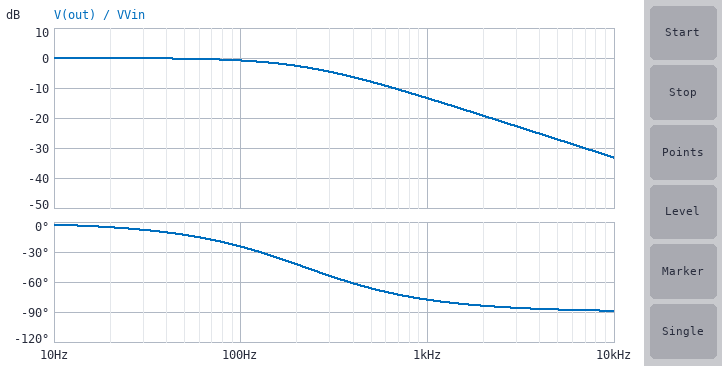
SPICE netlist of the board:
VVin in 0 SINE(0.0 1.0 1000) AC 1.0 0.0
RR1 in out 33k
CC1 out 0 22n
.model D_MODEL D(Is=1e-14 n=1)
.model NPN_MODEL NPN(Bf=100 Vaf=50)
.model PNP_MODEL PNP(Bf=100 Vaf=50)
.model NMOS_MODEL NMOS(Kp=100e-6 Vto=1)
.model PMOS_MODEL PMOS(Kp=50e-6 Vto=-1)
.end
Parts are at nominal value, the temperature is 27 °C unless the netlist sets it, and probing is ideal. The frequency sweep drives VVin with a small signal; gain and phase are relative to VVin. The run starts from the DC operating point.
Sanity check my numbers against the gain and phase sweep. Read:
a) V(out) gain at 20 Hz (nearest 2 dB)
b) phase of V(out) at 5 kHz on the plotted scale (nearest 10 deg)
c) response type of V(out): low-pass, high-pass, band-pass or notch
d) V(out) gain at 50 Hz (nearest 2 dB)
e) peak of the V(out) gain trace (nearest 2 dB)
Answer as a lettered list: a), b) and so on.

a) 0 dB
b) -90 deg
c) low-pass
d) 0 dB
e) 0 dB
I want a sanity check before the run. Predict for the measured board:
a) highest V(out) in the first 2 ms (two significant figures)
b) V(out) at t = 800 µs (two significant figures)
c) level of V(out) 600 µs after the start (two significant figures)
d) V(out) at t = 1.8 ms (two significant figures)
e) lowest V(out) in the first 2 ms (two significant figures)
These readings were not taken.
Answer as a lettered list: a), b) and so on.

a) 330 mV
b) -39 mV
c) 230 mV
d) -91 mV
e) -200 mV
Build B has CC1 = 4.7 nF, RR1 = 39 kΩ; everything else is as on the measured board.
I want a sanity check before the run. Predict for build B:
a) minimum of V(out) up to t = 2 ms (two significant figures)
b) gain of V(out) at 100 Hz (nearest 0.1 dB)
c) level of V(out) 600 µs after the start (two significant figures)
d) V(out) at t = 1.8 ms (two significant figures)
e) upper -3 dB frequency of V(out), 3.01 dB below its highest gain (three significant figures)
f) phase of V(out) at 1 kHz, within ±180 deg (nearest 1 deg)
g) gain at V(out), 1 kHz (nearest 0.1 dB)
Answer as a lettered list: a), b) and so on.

a) -660 mV
b) -0.1 dB
c) 170 mV
d) -560 mV
e) 868 Hz
f) -49 deg
g) -3.7 dB
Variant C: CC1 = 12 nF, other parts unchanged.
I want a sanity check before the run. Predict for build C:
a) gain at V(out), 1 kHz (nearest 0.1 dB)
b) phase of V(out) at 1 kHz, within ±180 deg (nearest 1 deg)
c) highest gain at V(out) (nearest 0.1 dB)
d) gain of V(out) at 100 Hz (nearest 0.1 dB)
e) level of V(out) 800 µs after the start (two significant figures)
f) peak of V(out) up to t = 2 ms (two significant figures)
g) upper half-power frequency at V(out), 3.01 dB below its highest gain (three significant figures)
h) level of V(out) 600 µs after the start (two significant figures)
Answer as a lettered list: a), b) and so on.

a) -8.6 dB
b) -68 deg
c) 0 dB
d) -0.3 dB
e) -190 mV
f) 490 mV
g) 402 Hz
h) 270 mV
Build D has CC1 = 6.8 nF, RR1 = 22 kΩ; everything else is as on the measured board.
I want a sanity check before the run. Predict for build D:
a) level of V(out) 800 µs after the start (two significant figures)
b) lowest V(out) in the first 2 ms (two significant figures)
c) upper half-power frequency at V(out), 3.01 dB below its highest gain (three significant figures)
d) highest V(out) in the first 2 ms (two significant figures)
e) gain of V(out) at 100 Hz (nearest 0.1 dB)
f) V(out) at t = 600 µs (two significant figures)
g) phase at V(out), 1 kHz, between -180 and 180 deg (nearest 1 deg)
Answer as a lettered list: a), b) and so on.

a) -660 mV
b) -730 mV
c) 1.06 kHz
d) 770 mV
e) 0 dB
f) 100 mV
g) -43 deg
